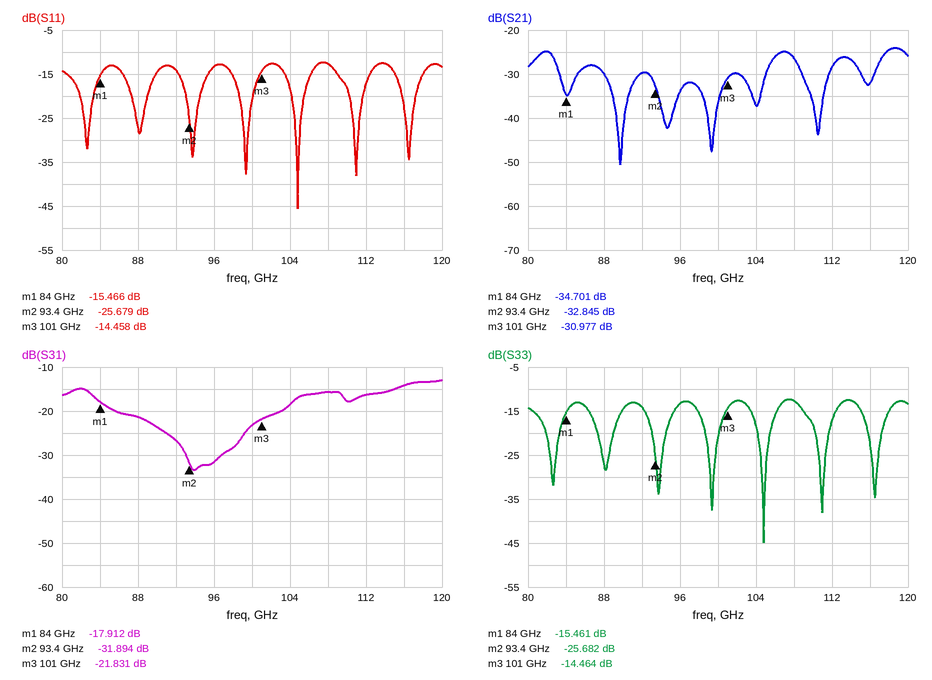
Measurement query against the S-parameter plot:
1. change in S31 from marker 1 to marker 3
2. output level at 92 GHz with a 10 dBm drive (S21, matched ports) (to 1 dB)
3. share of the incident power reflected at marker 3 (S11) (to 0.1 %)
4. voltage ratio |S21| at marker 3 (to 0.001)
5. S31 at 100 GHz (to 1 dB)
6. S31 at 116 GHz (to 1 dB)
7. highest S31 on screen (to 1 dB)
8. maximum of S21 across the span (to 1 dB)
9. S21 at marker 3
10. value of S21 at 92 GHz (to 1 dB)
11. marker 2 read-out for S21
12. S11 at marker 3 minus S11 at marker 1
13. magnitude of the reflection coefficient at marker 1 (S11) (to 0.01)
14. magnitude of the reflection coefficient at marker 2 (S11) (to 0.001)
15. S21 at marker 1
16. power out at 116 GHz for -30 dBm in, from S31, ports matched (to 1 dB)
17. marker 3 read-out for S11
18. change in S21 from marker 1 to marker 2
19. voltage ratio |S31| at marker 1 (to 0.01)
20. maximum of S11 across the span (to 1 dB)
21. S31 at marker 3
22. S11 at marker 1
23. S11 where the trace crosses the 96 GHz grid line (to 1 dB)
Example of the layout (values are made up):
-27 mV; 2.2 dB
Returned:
-3.919 dB; -20 dBm; 3.6 %; 0.028; -23 dB; -14 dB; -13 dB; -24 dB; -30.977 dB; -30 dB; -32.845 dB; 1.008 dB; 0.17; 0.052; -34.701 dB; -44 dBm; -14.458 dB; 1.856 dB; 0.13; -12 dB; -21.831 dB; -15.466 dB; -13 dB
